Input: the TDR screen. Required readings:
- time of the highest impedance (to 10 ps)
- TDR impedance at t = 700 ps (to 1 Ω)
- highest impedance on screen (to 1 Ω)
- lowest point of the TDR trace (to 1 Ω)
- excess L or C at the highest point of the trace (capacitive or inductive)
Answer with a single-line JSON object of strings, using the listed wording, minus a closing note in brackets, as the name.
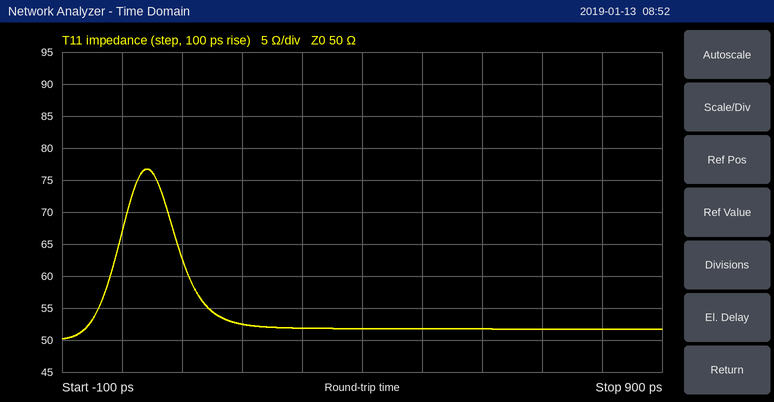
{"time of the highest impedance": "40 ps", "TDR impedance at t = 700 ps": "52 Ω", "highest impedance on screen": "77 Ω", "lowest point of the TDR trace": "50 Ω", "excess L or C at the highest point of the trace": "inductive"}
